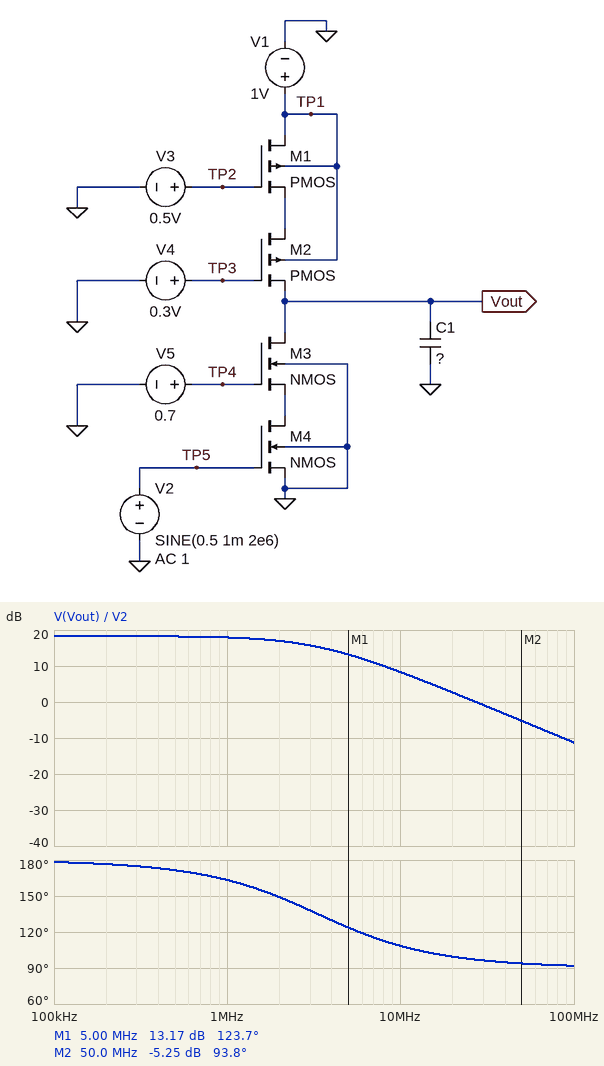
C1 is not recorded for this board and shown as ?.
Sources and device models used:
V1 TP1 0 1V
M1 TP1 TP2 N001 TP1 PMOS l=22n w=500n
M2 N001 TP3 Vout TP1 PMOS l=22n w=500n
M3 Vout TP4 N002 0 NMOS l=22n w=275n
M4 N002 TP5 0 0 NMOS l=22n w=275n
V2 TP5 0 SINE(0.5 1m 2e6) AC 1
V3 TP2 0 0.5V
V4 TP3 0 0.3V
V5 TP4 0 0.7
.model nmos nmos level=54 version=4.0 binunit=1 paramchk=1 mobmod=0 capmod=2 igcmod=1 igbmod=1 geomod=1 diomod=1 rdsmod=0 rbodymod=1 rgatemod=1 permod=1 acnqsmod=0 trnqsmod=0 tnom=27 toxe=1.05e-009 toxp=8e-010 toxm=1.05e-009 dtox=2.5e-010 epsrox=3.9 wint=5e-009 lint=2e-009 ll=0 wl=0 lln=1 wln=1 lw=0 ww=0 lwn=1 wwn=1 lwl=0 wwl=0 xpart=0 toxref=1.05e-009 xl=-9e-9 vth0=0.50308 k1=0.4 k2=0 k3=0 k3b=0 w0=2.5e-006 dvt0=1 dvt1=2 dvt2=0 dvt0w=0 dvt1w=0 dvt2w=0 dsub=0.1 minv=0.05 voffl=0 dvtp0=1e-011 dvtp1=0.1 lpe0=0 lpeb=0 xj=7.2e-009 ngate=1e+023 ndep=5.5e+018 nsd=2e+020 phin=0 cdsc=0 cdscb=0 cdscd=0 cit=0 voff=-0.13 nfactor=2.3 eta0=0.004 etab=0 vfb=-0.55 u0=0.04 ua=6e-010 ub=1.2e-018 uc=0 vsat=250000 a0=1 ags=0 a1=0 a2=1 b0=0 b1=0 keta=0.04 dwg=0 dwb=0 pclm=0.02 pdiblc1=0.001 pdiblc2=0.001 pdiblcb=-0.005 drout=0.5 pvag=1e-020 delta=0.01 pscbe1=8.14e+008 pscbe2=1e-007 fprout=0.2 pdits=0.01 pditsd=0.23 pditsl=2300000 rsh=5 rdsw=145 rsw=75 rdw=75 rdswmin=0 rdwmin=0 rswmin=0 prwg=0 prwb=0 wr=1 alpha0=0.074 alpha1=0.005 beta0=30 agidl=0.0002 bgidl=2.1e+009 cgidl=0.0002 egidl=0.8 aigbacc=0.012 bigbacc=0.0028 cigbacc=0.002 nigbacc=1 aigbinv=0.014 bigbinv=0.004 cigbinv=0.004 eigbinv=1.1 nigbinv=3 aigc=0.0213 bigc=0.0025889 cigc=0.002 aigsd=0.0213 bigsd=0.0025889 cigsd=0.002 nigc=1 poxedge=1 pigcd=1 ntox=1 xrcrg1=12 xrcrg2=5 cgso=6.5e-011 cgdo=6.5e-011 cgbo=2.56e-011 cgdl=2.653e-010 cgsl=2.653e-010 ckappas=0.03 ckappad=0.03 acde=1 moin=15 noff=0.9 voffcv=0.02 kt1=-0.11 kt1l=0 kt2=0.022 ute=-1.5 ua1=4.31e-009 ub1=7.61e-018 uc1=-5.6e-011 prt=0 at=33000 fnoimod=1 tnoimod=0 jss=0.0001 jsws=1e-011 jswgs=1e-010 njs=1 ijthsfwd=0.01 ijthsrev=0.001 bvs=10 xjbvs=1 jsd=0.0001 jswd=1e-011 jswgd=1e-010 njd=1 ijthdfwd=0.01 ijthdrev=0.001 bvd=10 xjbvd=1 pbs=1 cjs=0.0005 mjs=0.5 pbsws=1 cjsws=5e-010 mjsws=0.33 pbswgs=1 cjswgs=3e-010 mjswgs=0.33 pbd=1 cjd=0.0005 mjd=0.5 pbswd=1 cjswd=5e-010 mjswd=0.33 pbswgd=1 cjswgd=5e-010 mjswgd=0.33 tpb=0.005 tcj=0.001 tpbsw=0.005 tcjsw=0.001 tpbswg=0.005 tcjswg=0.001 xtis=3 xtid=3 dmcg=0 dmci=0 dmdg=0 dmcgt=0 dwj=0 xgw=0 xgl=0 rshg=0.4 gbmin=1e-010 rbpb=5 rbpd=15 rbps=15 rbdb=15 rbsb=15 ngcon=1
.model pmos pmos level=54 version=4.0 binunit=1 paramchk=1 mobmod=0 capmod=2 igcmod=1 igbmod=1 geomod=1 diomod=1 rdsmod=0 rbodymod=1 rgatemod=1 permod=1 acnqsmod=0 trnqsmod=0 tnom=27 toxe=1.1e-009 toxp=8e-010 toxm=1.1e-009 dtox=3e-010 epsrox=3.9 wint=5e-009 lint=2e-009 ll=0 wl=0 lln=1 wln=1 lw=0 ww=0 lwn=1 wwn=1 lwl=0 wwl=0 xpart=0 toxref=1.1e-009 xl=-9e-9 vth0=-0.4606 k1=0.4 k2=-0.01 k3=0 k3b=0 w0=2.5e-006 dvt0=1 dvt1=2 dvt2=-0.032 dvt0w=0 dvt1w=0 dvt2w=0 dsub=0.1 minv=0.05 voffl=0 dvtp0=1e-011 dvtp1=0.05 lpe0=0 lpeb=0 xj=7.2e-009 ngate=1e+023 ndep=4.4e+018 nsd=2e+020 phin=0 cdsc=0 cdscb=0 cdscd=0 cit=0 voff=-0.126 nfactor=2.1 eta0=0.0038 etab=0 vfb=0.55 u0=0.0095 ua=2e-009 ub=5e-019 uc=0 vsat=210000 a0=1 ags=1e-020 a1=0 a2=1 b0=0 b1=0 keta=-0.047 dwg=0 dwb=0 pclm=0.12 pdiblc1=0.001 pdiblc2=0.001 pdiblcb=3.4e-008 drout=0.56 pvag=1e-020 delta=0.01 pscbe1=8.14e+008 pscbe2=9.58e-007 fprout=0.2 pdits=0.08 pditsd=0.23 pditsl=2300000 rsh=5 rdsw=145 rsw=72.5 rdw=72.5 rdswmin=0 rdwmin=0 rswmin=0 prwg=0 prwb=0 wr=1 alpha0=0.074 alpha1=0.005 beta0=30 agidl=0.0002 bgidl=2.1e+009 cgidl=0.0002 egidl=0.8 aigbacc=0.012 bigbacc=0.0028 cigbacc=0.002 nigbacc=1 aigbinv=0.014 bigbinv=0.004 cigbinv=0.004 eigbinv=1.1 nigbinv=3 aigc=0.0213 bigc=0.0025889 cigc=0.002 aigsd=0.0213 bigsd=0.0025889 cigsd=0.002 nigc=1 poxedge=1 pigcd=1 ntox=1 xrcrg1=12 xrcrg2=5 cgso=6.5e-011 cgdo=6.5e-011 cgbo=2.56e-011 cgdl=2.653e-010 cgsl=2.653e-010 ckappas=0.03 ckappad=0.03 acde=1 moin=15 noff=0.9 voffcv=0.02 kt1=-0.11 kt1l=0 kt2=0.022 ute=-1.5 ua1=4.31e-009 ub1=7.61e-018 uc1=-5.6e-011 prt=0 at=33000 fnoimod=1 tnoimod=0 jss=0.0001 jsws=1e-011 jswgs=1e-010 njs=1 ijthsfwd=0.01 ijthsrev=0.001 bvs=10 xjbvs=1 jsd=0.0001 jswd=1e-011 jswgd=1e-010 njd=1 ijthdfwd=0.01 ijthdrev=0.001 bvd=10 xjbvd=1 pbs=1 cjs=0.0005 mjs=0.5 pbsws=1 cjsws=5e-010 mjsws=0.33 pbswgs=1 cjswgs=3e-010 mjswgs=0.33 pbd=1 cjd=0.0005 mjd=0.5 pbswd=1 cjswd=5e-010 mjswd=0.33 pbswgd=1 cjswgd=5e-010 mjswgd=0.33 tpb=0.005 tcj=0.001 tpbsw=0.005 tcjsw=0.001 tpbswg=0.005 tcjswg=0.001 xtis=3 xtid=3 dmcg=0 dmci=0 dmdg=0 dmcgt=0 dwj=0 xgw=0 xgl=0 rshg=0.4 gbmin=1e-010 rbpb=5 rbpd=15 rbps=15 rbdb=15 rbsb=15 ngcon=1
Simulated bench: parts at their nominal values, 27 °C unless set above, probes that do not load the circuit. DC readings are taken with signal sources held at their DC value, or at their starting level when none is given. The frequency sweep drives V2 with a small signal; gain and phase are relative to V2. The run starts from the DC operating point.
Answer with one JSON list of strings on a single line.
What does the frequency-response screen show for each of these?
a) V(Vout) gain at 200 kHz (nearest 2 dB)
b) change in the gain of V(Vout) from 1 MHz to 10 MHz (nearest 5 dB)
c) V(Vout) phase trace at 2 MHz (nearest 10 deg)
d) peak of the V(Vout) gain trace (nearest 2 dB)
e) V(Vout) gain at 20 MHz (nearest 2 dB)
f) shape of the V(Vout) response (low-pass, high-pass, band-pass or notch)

["18 dB", "-10 dB", "150 deg", "18 dB", "2 dB", "low-pass"]
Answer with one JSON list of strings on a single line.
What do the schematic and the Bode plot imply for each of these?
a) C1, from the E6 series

["2.2 pF"]
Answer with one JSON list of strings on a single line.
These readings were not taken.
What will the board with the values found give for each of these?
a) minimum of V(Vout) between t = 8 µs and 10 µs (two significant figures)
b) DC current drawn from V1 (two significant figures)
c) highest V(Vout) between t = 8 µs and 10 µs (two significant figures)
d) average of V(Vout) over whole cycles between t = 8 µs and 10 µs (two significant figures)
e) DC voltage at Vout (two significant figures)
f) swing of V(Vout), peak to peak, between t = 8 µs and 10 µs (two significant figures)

["510 mV", "38 µA", "520 mV", "520 mV", "520 mV", "14 mV"]
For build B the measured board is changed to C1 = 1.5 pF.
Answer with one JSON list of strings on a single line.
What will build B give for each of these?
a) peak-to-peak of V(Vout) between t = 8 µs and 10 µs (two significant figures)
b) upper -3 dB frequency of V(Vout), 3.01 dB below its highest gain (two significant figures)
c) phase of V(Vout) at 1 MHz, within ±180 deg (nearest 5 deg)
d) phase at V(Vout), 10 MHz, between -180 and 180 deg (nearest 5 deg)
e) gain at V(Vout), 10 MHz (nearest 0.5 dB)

["15 mV", "4.9 MHz", "170 deg", "115 deg", "11.0 dB"]
